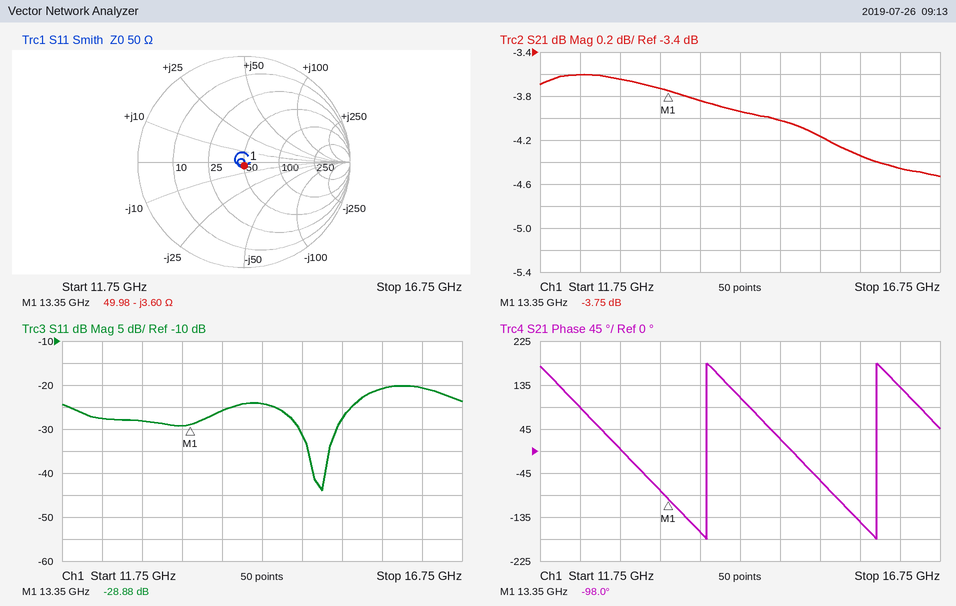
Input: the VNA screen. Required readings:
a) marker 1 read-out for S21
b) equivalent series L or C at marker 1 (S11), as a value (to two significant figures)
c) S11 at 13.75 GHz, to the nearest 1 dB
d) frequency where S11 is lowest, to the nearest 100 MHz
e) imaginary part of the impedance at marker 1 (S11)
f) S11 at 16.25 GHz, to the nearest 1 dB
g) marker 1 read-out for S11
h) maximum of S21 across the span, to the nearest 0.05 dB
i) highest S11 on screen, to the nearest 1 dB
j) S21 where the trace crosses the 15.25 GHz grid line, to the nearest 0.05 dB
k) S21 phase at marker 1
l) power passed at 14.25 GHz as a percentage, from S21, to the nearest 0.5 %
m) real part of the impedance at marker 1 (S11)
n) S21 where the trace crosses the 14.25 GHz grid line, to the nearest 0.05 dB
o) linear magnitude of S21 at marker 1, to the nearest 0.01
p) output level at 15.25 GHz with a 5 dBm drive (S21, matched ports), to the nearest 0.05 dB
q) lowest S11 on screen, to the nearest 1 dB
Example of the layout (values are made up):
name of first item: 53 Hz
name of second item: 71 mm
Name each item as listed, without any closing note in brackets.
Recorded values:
marker 1 read-out for S21: -3.75 dB
equivalent series L or C at marker 1 (S11), as a value: 3.3 pF
S11 at 13.75 GHz, to the nearest 1 dB: -26 dB
frequency where S11 is lowest, to the nearest 100 MHz: 15.0 GHz
imaginary part of the impedance at marker 1: -3.60 Ω
S11 at 16.25 GHz, to the nearest 1 dB: -21 dB
marker 1 read-out for S11: -28.88 dB
maximum of S21 across the span, to the nearest 0.05 dB: -3.60 dB
highest S11 on screen, to the nearest 1 dB: -20 dB
S21 where the trace crosses the 15.25 GHz grid line, to the nearest 0.05 dB: -4.15 dB
S21 phase at marker 1: -98.0°
power passed at 14.25 GHz as a percentage, from S21, to the nearest 0.5 %: 40.5 %
real part of the impedance at marker 1: 49.98 Ω
S21 where the trace crosses the 14.25 GHz grid line, to the nearest 0.05 dB: -3.95 dB
linear magnitude of S21 at marker 1, to the nearest 0.01: 0.65
output level at 15.25 GHz with a 5 dBm drive (S21, matched ports), to the nearest 0.05 dB: 0.85 dBm
lowest S11 on screen, to the nearest 1 dB: -44 dB
